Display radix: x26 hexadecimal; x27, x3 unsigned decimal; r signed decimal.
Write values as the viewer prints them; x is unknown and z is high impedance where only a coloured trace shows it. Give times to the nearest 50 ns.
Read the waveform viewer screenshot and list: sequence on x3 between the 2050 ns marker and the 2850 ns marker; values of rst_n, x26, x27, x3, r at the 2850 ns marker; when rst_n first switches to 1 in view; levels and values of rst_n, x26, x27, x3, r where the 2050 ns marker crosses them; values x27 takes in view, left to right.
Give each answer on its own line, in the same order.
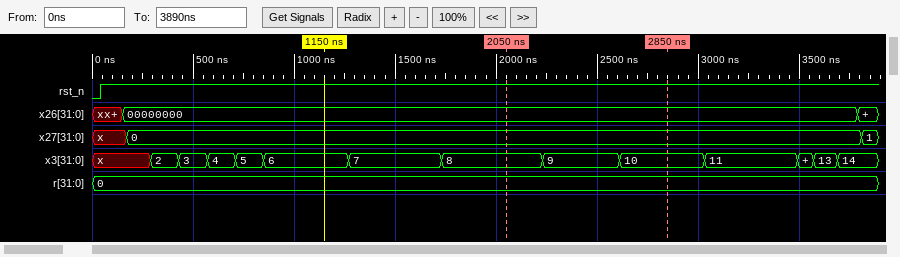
8, 9, 10
rst_n=1, x26=00000000, x27=0, x3=10, r=0
50 ns
rst_n=1, x26=00000000, x27=0, x3=8, r=0
x, 0, 1
